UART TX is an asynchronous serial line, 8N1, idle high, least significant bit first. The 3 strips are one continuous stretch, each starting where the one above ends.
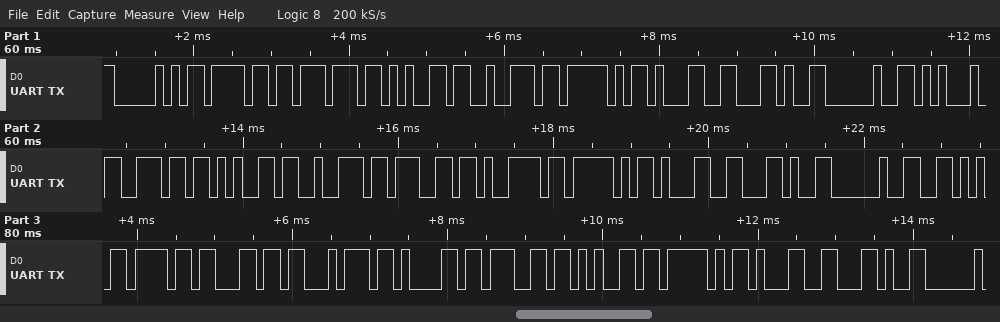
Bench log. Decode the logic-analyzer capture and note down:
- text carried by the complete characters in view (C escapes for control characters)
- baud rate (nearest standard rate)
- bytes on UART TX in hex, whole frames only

"Power_1, Energy_1, Voltage_1,"
9600 baud
50 6F 77 65 72 5F 31 2C 20 45 6E 65 72 67 79 5F 31 2C 20 56 6F 6C 74 61 67 65 5F 31 2C
